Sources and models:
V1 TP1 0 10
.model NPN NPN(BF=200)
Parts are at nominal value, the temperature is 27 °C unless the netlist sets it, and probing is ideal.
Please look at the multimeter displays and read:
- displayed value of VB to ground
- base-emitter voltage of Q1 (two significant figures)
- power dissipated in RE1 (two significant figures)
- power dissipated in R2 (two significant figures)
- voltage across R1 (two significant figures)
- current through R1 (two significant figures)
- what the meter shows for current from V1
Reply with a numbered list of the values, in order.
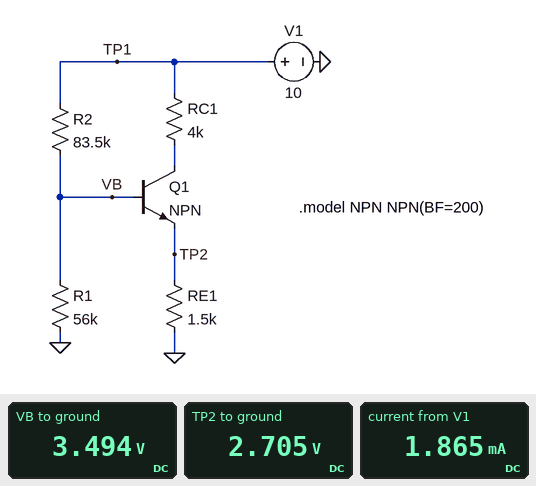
1. 3.494 V
2. 790 mV
3. 4.9 mW
4. 510 µW
5. 3.5 V
6. 62 µA
7. 1.865 mA
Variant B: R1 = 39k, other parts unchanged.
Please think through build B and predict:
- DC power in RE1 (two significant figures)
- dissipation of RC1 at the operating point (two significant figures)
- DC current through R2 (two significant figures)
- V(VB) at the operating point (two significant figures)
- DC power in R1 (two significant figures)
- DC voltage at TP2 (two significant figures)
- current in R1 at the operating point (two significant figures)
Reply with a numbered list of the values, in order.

1. 3.2 mW
2. 8.6 mW
3. 84 µA
4. 3.0 V
5. 230 µW
6. 2.2 V
7. 77 µA
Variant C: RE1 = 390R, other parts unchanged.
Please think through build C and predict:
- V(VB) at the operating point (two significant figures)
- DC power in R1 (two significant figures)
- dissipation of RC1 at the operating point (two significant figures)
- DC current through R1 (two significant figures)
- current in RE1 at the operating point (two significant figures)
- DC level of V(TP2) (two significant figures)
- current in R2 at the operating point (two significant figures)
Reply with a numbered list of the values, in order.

1. 1.7 V
2. 52 µW
3. 20 mW
4. 30 µA
5. 2.3 mA
6. 900 mV
7. 99 µA
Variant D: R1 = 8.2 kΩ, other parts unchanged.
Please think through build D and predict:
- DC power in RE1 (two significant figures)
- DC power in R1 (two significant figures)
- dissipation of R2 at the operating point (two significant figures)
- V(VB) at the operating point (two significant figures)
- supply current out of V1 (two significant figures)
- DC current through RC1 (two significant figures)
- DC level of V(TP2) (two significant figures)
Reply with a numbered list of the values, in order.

1. 20 µW
2. 97 µW
3. 990 µW
4. 890 mV
5. 220 µA
6. 110 µA
7. 170 mV
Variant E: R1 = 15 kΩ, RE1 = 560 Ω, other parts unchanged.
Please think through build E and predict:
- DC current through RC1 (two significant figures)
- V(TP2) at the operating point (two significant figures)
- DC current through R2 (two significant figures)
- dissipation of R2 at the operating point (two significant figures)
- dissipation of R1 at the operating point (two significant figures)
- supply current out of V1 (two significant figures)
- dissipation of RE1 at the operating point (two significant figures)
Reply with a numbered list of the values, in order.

1. 1.2 mA
2. 670 mV
3. 100 µA
4. 880 µW
5. 140 µW
6. 1.3 mA
7. 800 µW
